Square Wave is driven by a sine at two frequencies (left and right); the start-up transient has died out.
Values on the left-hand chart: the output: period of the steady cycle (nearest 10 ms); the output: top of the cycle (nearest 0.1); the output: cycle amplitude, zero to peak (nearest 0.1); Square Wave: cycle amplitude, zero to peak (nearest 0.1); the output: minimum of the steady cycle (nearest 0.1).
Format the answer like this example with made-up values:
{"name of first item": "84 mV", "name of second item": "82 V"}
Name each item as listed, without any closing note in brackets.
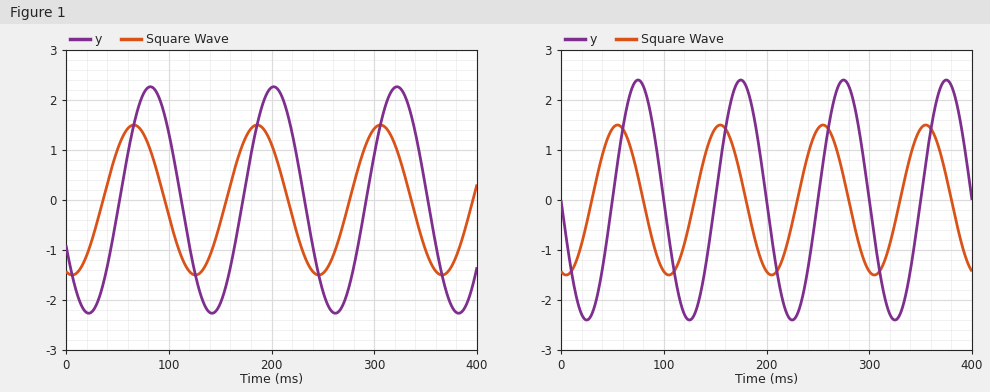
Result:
{"the output: period of the steady cycle": "120 ms", "the output: top of the cycle": "2.3", "the output: cycle amplitude, zero to peak": "2.3", "Square Wave: cycle amplitude, zero to peak": "1.5", "the output: minimum of the steady cycle": "-2.3"}
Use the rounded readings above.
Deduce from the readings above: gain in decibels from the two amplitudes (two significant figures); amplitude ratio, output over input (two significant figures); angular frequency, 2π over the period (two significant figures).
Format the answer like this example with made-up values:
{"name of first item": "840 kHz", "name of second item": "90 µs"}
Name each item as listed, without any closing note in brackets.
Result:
{"gain in decibels from the two amplitudes": "3.7 dB", "amplitude ratio, output over input": "1.5", "angular frequency, 2π over the period": "0.052 rad/ms"}
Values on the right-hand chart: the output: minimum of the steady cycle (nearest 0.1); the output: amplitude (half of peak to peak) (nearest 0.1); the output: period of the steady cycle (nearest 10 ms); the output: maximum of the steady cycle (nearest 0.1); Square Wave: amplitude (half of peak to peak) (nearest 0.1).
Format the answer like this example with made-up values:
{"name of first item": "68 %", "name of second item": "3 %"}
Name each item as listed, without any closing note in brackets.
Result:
{"the output: minimum of the steady cycle": "-2.4", "the output: amplitude (half of peak to peak)": "2.4", "the output: period of the steady cycle": "100 ms", "the output: maximum of the steady cycle": "2.4", "Square Wave: amplitude (half of peak to peak)": "1.5"}
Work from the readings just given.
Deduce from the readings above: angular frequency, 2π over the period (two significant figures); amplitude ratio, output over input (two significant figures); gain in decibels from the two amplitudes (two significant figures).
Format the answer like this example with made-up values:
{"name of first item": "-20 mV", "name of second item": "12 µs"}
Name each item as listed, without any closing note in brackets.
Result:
{"angular frequency, 2π over the period": "0.063 rad/ms", "amplitude ratio, output over input": "1.6", "gain in decibels from the two amplitudes": "4.1 dB"}
